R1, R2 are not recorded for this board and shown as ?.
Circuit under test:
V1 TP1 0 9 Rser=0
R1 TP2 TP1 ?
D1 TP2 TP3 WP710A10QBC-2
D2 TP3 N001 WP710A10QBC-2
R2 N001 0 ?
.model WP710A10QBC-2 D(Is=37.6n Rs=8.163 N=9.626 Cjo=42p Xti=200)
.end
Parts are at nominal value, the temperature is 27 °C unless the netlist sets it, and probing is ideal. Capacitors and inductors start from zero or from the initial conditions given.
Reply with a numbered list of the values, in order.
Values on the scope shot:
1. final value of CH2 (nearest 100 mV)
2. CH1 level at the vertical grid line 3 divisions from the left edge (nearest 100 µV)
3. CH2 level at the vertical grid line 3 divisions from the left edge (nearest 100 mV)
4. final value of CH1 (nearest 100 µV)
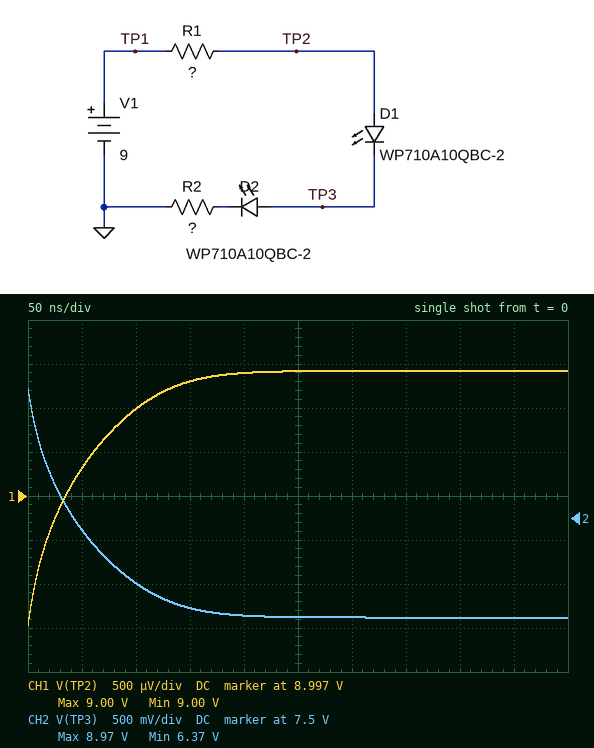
1. 6.4 V
2. 8.9978 V
3. 6.5 V
4. 8.9979 V
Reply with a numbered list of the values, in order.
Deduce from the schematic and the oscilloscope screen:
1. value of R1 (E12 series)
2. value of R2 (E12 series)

1. 1.5 Ω
2. 2.7 kΩ
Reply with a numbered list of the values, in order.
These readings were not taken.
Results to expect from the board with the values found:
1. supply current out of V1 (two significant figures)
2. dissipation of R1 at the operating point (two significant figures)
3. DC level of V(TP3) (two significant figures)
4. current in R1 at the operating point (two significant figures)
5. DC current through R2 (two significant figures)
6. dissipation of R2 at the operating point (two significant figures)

1. 1.4 mA
2. 2.9 µW
3. 6.4 V
4. 1.4 mA
5. 1.4 mA
6. 5.2 mW
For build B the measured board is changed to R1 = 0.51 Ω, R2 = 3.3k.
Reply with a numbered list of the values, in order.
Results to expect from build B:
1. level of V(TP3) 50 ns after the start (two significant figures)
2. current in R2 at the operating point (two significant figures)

1. 7.5 V
2. 1.2 mA
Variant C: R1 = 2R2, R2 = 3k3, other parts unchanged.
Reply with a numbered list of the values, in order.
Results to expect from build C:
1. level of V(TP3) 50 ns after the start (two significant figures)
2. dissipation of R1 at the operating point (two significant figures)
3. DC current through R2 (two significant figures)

1. 7.5 V
2. 3.0 µW
3. 1.2 mA
